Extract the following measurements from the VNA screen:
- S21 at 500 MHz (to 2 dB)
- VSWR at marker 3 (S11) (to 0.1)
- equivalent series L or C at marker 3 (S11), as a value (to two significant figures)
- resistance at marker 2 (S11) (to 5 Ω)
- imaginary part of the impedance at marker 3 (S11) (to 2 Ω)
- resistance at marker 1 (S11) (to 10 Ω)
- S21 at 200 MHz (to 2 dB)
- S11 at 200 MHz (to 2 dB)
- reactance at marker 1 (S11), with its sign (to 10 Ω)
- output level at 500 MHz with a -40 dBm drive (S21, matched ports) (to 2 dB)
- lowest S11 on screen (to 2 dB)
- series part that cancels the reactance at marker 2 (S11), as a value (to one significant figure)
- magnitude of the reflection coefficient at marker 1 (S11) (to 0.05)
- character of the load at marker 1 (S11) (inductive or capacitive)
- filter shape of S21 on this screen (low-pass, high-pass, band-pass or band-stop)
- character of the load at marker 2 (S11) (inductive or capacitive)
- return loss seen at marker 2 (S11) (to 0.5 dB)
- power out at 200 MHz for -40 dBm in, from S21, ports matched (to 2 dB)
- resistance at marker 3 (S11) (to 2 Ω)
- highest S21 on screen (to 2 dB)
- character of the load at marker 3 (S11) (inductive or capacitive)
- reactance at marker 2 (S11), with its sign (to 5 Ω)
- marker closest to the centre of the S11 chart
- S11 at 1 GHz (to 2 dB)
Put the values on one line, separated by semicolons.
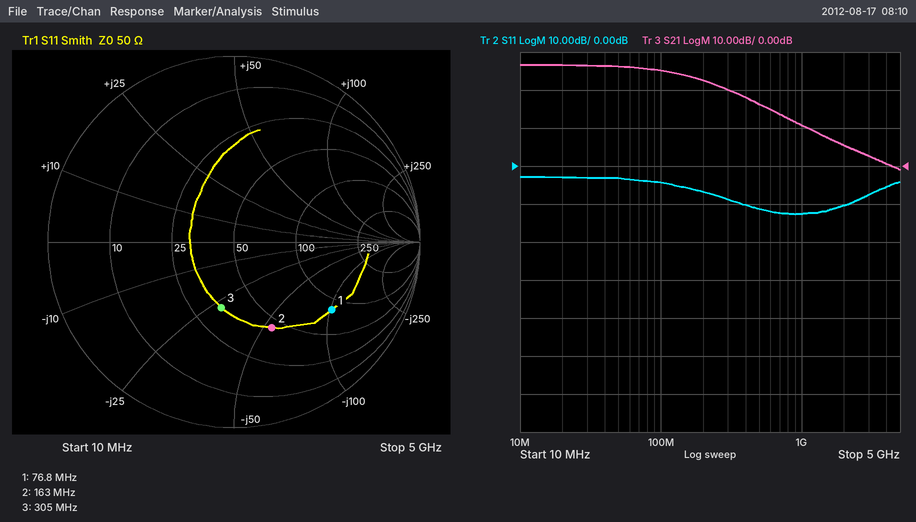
16 dB; 2.1; 19 pF; 45 Ω; -28 Ω; 80 Ω; 22 dB; -6 dB; -100 Ω; -24 dBm; -12 dB; 50 nH; 0.65; capacitive; low-pass; capacitive; 6.0 dB; -18 dBm; 34 Ω; 26 dB; capacitive; -55 Ω; marker 3; -12 dB
